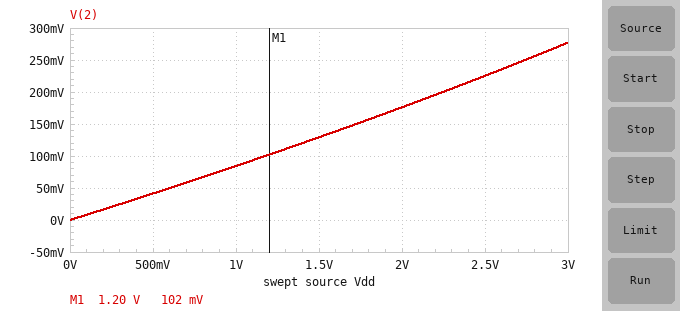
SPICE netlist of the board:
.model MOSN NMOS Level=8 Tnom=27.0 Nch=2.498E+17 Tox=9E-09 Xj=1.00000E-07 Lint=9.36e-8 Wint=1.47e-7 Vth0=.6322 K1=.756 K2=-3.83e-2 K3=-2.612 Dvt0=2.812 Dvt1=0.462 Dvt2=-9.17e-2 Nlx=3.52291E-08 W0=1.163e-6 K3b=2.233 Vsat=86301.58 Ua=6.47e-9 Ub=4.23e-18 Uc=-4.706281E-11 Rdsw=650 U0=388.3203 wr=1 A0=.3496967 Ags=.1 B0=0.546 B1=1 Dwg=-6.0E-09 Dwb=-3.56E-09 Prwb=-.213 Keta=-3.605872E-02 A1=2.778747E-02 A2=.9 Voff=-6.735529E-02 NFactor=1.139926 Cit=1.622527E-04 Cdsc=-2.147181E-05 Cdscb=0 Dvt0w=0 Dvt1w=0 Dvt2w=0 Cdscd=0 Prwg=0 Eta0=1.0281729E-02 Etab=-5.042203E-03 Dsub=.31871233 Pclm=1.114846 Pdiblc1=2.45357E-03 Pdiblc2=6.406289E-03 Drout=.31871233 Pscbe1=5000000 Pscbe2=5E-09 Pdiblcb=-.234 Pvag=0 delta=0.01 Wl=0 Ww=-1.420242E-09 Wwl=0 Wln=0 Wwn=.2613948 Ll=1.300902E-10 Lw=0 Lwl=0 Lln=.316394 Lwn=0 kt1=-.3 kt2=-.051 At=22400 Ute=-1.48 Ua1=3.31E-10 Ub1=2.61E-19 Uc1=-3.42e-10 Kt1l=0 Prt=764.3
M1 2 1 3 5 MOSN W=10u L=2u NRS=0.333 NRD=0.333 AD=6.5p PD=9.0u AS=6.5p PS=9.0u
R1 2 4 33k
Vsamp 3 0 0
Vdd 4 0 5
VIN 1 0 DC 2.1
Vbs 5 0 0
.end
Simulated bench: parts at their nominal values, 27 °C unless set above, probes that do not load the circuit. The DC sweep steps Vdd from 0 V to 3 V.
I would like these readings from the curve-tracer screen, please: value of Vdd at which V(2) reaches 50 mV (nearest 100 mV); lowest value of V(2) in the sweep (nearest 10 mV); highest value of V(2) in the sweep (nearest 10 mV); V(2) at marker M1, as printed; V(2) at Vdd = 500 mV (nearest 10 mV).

600 mV
0 V
280 mV
102 mV
40 mV
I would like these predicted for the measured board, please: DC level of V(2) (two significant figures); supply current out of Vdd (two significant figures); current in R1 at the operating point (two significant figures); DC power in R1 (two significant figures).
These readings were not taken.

520 mV
140 µA
140 µA
610 µW
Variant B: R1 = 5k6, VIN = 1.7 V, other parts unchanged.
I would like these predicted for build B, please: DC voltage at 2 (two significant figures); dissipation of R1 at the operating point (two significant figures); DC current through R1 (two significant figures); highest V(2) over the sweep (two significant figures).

4.3 V
84 µW
120 µA
2.3 V
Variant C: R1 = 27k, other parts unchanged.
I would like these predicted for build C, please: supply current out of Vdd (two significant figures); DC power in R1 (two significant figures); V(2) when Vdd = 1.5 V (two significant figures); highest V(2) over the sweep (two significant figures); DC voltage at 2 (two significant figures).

160 µA
690 µW
160 mV
340 mV
680 mV
